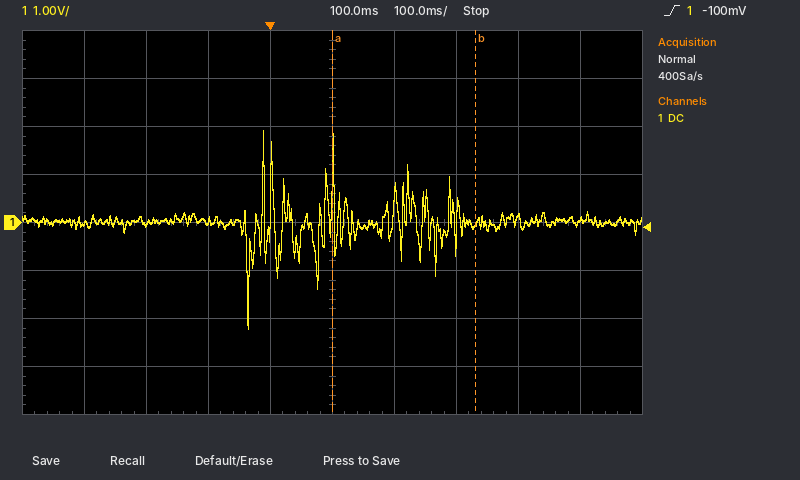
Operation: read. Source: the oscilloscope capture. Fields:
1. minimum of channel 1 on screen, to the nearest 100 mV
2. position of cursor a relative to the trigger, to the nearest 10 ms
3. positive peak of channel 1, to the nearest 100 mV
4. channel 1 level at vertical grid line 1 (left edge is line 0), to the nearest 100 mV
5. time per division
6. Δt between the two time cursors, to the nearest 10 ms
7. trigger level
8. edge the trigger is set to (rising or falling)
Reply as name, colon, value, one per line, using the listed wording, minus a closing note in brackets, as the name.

minimum of channel 1 on screen, to the nearest 100 mV: -2.2 V
position of cursor a relative to the trigger, to the nearest 10 ms: +100 ms
positive peak of channel 1, to the nearest 100 mV: 1.9 V
channel 1 level at vertical grid line 1 (left edge is line 0), to the nearest 100 mV: 0.0 V
time per division: 100 ms
Δt between the two time cursors, to the nearest 10 ms: 230 ms
trigger level: -100 mV
edge the trigger is set to: rising
